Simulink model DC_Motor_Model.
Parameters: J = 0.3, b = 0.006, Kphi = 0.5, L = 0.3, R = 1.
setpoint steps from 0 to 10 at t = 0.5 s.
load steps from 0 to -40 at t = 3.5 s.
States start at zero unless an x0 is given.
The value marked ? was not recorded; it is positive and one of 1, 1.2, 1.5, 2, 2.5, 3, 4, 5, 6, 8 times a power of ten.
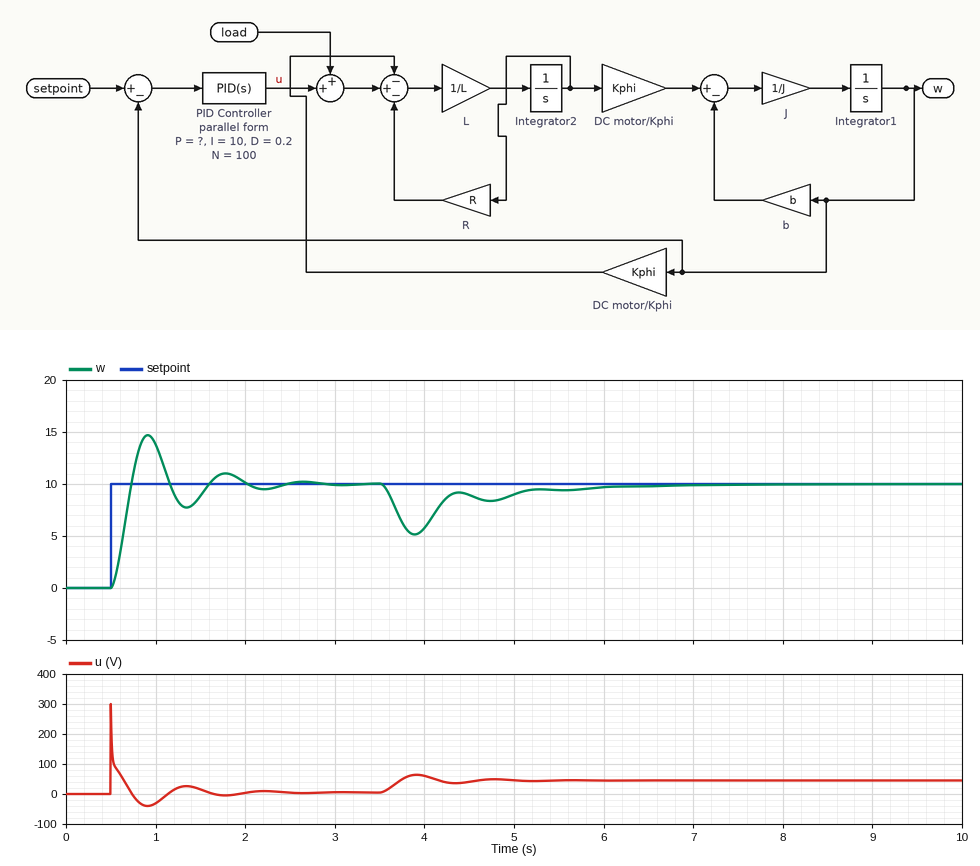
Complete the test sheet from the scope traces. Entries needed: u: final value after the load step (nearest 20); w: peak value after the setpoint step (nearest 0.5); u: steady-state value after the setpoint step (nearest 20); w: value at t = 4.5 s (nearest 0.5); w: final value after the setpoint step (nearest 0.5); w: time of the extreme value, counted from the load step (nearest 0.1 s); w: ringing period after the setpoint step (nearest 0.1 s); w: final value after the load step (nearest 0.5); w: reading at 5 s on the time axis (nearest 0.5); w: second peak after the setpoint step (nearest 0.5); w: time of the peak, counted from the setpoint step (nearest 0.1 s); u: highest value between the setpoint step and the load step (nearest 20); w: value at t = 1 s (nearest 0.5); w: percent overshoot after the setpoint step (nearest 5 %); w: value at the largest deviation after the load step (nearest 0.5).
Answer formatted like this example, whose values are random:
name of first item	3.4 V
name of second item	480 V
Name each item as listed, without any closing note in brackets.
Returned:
u: final value after the load step	40
w: peak value after the setpoint step	14.5
u: steady-state value after the setpoint step	0
w: value at t = 4.5 s	9.0
w: final value after the setpoint step	10.0
w: time of the extreme value, counted from the load step	0.4 s
w: ringing period after the setpoint step	0.9 s
w: final value after the load step	10.0
w: reading at 5 s on the time axis	9.0
w: second peak after the setpoint step	11.0
w: time of the peak, counted from the setpoint step	0.4 s
u: highest value between the setpoint step and the load step	300
w: value at t = 1 s	14.0
w: percent overshoot after the setpoint step	45 %
w: value at the largest deviation after the load step	5.0
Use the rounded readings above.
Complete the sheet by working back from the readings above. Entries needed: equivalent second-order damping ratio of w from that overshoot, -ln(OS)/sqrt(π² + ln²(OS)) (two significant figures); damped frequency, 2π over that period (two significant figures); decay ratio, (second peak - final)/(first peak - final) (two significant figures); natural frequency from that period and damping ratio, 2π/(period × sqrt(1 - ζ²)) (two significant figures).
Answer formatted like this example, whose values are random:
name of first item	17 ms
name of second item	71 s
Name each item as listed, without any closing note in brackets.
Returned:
equivalent second-order damping ratio of w from that overshoot, -ln(OS)/sqrt(π² + ln²(OS))	0.25
damped frequency, 2π over that period	7.0 rad/s
decay ratio, (second peak - final)/(first peak - final)	0.22
natural frequency from that period and damping ratio, 2π/(period × sqrt(1 - ζ²))	7.2 rad/s
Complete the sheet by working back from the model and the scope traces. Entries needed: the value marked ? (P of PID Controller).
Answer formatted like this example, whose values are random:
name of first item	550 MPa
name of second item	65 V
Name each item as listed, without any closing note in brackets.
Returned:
the value marked ?	10
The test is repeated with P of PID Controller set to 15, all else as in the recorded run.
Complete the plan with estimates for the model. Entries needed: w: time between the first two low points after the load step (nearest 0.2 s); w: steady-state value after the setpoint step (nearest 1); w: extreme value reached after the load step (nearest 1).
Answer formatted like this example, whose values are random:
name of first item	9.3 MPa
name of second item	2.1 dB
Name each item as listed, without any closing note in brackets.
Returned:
w: time between the first two low points after the load step	0.6 s
w: steady-state value after the setpoint step	10
w: extreme value reached after the load step	6
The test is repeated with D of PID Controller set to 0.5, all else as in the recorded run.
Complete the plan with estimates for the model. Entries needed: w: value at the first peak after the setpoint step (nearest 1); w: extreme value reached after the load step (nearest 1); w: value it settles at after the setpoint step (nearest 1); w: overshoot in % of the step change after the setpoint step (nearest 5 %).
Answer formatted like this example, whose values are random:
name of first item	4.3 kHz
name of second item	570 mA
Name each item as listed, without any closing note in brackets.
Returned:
w: value at the first peak after the setpoint step	13
w: extreme value reached after the load step	6
w: value it settles at after the setpoint step	10
w: overshoot in % of the step change after the setpoint step	35 %
